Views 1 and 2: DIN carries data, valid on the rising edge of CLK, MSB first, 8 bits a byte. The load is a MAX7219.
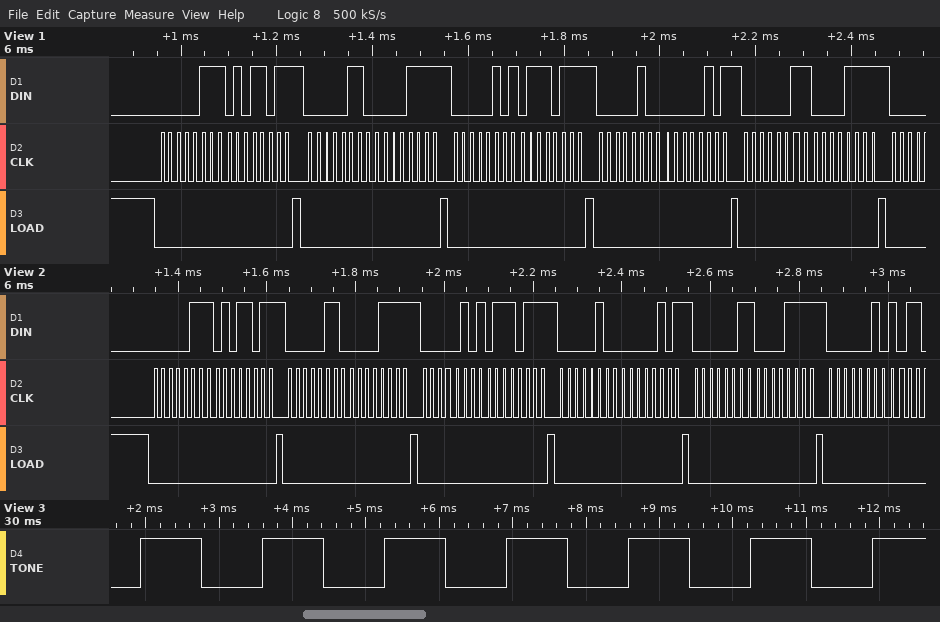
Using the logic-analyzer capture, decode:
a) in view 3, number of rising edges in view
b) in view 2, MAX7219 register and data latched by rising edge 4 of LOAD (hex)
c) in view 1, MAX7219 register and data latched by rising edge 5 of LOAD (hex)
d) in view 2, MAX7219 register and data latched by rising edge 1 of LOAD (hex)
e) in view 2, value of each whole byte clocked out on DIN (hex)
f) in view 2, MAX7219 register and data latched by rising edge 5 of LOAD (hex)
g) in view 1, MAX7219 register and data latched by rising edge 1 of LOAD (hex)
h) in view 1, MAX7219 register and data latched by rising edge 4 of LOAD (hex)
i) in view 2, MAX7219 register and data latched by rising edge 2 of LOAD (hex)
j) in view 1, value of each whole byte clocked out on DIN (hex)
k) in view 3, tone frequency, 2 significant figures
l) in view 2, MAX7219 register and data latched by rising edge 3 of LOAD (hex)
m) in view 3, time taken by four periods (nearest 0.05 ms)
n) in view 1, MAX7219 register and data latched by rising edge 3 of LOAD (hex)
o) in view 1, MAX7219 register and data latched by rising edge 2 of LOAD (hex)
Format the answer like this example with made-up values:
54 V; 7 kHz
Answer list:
7; register 0x4, data 0x05; register 0x3, data 0x0F; register 0x7, data 0x5B; 07 5B 06 0F 05 77 04 05 03 0F 02; register 0x3, data 0x0F; register 0x7, data 0x5B; register 0x4, data 0x05; register 0x6, data 0x0F; 0x07 0x5B 0x06 0x0F 0x05 0x77 0x04 0x05 0x03 0x0F; 600 Hz; register 0x5, data 0x77; 6.65 ms; register 0x5, data 0x77; register 0x6, data 0x0F
